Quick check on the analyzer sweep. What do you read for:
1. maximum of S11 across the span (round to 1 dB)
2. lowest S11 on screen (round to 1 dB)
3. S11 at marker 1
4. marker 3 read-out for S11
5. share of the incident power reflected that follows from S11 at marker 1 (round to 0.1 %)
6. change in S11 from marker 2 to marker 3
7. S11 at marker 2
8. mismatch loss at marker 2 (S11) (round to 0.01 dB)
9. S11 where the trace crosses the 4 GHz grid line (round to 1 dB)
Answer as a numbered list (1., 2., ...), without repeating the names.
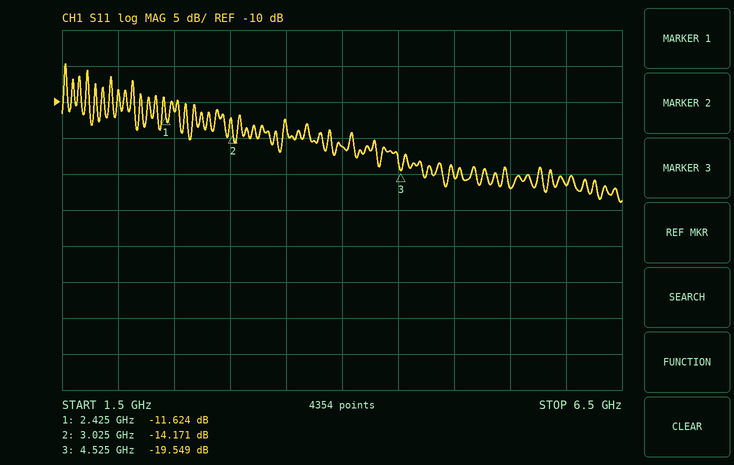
1. -5 dB
2. -24 dB
3. -11.624 dB
4. -19.549 dB
5. 6.9 %
6. -5.378 dB
7. -14.171 dB
8. 0.17 dB
9. -16 dB
